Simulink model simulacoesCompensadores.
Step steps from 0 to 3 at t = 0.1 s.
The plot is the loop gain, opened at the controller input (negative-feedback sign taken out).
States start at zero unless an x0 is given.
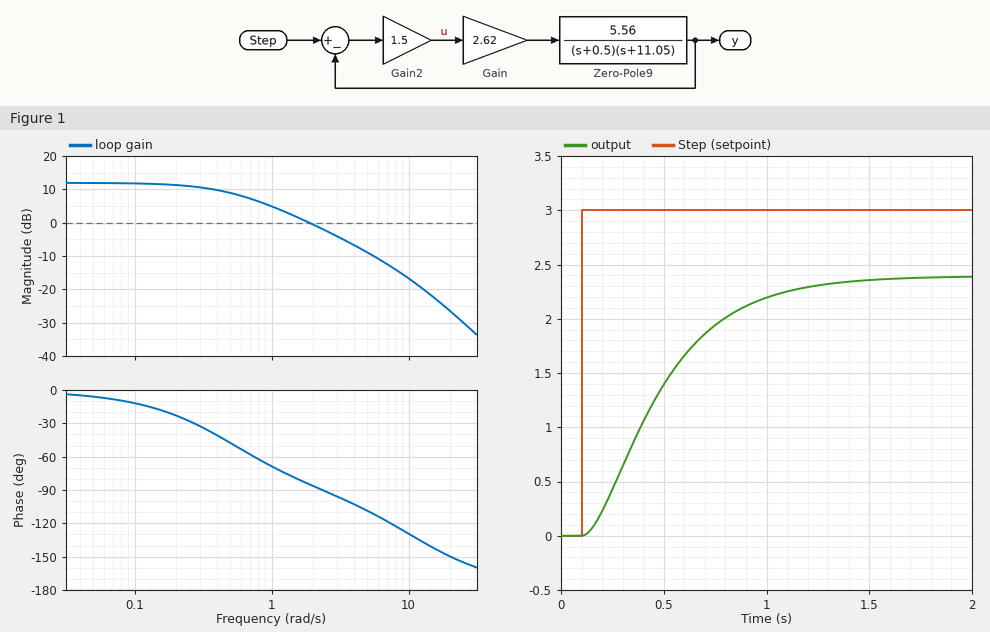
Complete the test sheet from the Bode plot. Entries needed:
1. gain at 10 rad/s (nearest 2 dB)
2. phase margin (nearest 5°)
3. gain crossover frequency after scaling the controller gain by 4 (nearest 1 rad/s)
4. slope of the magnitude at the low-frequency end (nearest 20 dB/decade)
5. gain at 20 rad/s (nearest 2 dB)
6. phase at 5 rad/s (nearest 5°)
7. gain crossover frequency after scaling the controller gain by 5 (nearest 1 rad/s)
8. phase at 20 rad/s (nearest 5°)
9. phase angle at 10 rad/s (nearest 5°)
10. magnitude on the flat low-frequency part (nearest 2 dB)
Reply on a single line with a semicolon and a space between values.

-16 dB; 95°; 7 rad/s; 0 dB/decade; -26 dB; -110°; 8 rad/s; -150°; -130°; 12 dB
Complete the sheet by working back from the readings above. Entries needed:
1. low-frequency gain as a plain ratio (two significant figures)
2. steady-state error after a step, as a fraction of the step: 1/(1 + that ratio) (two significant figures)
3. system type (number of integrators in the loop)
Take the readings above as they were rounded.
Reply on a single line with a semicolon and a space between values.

4.0; 0.20; 0
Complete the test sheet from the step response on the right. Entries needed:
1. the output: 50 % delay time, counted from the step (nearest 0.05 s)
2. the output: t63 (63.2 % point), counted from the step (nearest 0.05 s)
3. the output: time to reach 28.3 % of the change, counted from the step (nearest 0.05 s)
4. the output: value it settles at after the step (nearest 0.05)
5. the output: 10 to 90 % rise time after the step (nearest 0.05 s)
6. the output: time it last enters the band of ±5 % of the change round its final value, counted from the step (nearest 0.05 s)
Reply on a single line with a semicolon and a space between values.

0.35 s; 0.45 s; 0.20 s; 2.40; 0.75 s; 1.05 s
